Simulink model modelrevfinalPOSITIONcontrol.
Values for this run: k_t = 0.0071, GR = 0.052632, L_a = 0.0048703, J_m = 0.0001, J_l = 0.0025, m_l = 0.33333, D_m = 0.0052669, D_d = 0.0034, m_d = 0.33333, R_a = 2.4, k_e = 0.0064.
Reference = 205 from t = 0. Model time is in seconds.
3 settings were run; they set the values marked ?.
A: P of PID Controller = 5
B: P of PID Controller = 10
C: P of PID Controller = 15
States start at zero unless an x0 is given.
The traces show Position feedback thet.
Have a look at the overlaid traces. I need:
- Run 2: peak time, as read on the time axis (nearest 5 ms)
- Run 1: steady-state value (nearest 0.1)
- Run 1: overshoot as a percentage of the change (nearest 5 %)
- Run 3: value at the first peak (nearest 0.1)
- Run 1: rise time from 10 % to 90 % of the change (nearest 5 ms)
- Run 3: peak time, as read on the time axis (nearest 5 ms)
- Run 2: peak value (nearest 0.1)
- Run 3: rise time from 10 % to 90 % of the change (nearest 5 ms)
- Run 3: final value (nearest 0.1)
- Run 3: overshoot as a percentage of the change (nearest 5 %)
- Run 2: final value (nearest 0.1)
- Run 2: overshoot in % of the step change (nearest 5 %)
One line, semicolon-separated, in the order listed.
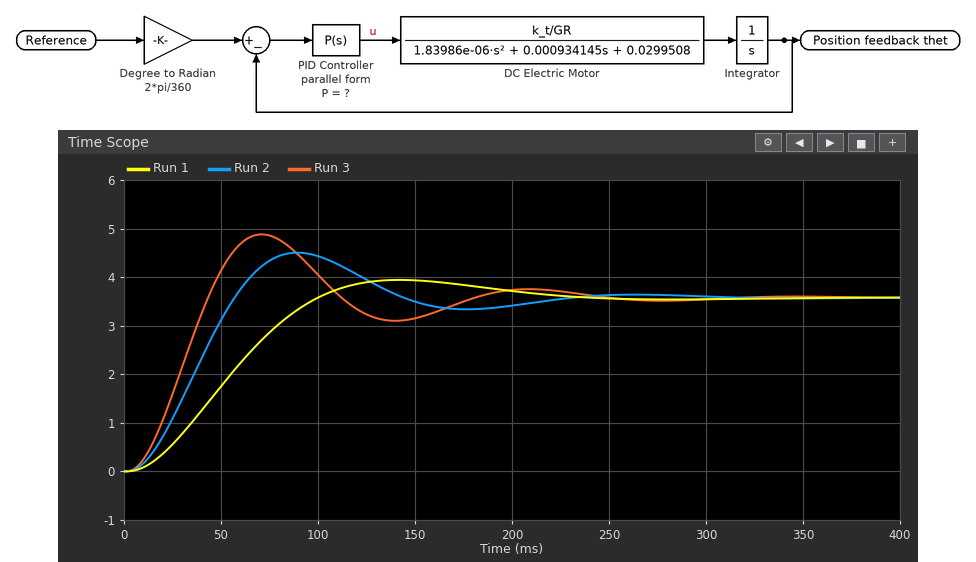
90 ms; 3.6; 10 %; 4.9; 65 ms; 70 ms; 4.5; 30 ms; 3.6; 35 %; 3.6; 25 %
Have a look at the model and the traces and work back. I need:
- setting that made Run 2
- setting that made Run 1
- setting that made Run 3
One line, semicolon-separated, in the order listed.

B; A; C
